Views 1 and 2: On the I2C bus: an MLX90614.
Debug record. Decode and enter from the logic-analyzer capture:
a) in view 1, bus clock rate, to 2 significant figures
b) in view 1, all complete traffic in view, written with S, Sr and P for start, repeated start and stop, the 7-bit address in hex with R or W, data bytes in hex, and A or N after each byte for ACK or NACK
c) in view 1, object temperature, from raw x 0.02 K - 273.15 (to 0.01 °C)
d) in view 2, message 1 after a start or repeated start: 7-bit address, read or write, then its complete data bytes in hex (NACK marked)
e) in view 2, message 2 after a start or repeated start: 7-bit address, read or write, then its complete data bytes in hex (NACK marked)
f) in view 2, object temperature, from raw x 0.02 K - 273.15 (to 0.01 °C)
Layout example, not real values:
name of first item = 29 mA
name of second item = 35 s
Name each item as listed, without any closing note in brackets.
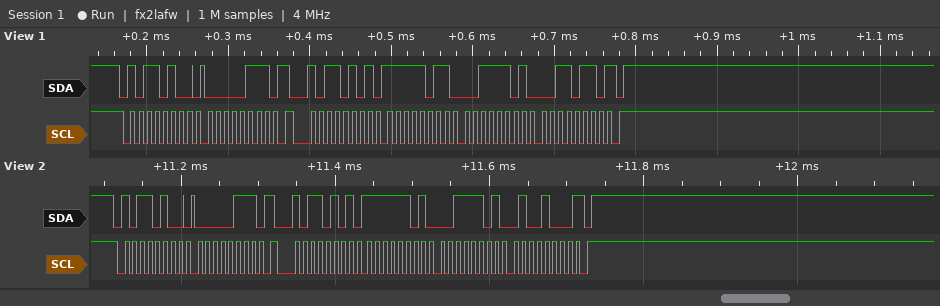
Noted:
in view 1, bus clock rate, to 2 significant figures = 100 kHz
in view 1, all complete traffic in view, written with S, Sr and P for start, repeated start and stop, the 7-bit address in hex with R or W, data bytes in hex, and A or N after each byte for ACK or NACK = S 5AW A 07 A Sr 5AR A FB A 3D A 36 N P
in view 1, object temperature, from raw x 0.02 K - 273.15 = 44.19 °C
in view 2, message 1 after a start or repeated start: 7-bit address, read or write, then its complete data bytes in hex = 0x5A write: 07
in view 2, message 2 after a start or repeated start: 7-bit address, read or write, then its complete data bytes in hex = 0x5A read: FD 3D 48 NACK
in view 2, object temperature, from raw x 0.02 K - 273.15 = 44.23 °C
